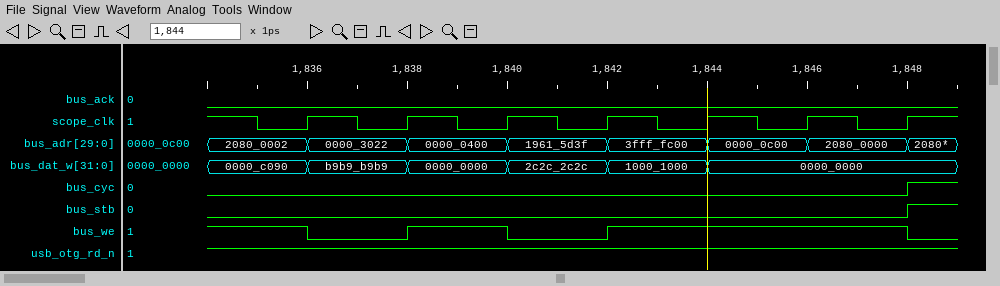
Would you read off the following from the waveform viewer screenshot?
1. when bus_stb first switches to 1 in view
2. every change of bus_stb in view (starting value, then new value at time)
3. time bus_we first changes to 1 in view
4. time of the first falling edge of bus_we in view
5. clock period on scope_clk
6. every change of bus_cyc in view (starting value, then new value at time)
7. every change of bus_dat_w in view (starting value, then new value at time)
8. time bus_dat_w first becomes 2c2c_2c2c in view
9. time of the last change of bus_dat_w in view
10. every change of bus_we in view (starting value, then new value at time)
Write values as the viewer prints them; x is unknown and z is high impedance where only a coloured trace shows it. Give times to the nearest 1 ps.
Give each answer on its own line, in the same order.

1848 ps
0, 1 at 1848 ps
1838 ps
1836 ps
2 ps
0, 1 at 1848 ps
0000_c090, b9b9_b9b9 at 1836 ps, 0000_0000 at 1838 ps, 2c2c_2c2c at 1840 ps, 1000_1000 at 1842 ps, 0000_0000 at 1844 ps
1840 ps
1844 ps
1, 0 at 1836 ps, 1 at 1838 ps, 0 at 1840 ps, 1 at 1842 ps, 0 at 1848 ps
